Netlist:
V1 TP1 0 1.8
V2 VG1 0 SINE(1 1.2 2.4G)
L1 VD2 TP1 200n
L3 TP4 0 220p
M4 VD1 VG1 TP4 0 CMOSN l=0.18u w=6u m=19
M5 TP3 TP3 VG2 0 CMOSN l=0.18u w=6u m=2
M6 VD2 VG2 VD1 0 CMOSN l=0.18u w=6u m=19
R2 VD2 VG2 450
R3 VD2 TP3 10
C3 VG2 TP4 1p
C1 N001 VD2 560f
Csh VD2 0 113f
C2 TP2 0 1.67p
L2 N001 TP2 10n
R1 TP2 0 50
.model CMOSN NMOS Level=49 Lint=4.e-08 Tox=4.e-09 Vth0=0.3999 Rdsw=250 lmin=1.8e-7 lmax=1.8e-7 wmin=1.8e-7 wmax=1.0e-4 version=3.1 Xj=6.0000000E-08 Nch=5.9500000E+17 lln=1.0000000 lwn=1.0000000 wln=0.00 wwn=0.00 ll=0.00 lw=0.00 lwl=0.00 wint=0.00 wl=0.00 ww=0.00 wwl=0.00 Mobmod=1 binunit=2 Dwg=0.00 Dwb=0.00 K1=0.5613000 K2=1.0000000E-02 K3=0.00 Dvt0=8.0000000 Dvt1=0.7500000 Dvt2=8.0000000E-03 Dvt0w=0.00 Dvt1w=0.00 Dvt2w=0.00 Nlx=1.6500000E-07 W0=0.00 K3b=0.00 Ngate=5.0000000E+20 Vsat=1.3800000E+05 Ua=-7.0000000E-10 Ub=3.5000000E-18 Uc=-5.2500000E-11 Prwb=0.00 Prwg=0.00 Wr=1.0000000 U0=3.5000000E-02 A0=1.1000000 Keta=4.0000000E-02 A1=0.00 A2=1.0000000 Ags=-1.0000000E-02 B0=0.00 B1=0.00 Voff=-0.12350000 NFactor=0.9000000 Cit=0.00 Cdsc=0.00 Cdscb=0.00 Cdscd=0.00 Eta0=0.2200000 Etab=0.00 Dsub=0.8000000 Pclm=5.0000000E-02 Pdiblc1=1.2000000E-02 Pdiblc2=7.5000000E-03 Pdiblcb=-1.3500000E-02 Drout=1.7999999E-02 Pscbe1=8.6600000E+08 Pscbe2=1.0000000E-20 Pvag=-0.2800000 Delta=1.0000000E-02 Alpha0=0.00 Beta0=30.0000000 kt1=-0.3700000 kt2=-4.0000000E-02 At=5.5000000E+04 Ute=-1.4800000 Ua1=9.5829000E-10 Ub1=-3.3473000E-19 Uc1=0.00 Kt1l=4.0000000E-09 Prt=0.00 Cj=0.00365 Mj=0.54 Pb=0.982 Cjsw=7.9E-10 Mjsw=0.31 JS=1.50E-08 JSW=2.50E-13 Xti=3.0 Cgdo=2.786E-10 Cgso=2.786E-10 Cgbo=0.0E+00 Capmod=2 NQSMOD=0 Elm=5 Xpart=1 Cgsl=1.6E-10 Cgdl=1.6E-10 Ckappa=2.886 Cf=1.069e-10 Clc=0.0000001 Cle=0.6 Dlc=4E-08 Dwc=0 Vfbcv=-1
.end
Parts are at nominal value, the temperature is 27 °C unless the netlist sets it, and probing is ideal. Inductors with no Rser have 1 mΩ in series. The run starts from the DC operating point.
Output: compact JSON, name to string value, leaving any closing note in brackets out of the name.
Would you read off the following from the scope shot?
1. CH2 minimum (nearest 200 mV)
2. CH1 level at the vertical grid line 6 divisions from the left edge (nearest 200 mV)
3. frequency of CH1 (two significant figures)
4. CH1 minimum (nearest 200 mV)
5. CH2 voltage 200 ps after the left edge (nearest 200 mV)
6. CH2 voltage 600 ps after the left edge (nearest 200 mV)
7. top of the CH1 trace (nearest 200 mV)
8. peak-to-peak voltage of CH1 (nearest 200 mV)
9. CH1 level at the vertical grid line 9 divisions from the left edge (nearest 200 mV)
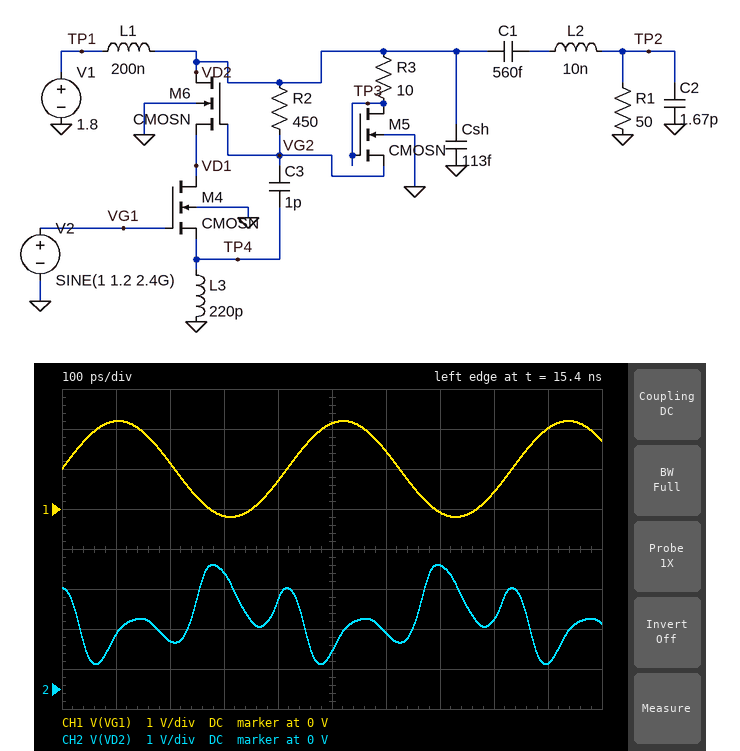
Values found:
{"CH2 minimum": "600 mV", "CH1 level at the vertical grid line 6 divisions from the left edge": "1.4 V", "frequency of CH1": "2.4 GHz", "CH1 minimum": "-200 mV", "CH2 voltage 200 ps after the left edge": "1.2 V", "CH2 voltage 600 ps after the left edge": "1.4 V", "top of the CH1 trace": "2.2 V", "peak-to-peak voltage of CH1": "2.4 V", "CH1 level at the vertical grid line 9 divisions from the left edge": "2.0 V"}
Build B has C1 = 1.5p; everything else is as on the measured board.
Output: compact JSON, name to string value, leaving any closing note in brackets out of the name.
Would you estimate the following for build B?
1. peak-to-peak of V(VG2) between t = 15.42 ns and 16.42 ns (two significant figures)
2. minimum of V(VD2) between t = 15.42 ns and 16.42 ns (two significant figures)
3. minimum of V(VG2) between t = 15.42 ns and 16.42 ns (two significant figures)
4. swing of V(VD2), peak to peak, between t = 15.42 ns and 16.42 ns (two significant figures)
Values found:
{"peak-to-peak of V(VG2) between t = 15.42 ns and 16.42 ns": "1.2 V", "minimum of V(VD2) between t = 15.42 ns and 16.42 ns": "-130 mV", "minimum of V(VG2) between t = 15.42 ns and 16.42 ns": "1.8 V", "swing of V(VD2), peak to peak, between t = 15.42 ns and 16.42 ns": "5.2 V"}
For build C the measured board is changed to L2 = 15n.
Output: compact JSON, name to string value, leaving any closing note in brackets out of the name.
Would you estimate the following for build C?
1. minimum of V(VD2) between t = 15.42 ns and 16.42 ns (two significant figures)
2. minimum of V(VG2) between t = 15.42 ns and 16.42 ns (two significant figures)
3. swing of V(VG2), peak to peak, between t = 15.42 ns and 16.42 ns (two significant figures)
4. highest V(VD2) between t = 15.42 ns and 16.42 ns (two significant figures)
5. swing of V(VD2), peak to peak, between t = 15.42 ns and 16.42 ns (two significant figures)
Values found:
{"minimum of V(VD2) between t = 15.42 ns and 16.42 ns": "-170 mV", "minimum of V(VG2) between t = 15.42 ns and 16.42 ns": "1.8 V", "swing of V(VG2), peak to peak, between t = 15.42 ns and 16.42 ns": "1.2 V", "highest V(VD2) between t = 15.42 ns and 16.42 ns": "5.0 V", "swing of V(VD2), peak to peak, between t = 15.42 ns and 16.42 ns": "5.1 V"}
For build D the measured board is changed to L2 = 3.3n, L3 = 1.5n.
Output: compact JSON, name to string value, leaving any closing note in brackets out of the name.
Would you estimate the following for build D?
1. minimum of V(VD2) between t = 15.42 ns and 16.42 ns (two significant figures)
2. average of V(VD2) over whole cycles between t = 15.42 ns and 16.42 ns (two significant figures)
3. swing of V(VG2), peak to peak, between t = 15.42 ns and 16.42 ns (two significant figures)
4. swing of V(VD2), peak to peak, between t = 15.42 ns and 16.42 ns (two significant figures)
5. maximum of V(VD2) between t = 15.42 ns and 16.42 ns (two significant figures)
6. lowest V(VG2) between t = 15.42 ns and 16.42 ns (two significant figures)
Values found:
{"minimum of V(VD2) between t = 15.42 ns and 16.42 ns": "-450 mV", "average of V(VD2) over whole cycles between t = 15.42 ns and 16.42 ns": "1.8 V", "swing of V(VG2), peak to peak, between t = 15.42 ns and 16.42 ns": "2.1 V", "swing of V(VD2), peak to peak, between t = 15.42 ns and 16.42 ns": "4.9 V", "maximum of V(VD2) between t = 15.42 ns and 16.42 ns": "4.4 V", "lowest V(VG2) between t = 15.42 ns and 16.42 ns": "980 mV"}
